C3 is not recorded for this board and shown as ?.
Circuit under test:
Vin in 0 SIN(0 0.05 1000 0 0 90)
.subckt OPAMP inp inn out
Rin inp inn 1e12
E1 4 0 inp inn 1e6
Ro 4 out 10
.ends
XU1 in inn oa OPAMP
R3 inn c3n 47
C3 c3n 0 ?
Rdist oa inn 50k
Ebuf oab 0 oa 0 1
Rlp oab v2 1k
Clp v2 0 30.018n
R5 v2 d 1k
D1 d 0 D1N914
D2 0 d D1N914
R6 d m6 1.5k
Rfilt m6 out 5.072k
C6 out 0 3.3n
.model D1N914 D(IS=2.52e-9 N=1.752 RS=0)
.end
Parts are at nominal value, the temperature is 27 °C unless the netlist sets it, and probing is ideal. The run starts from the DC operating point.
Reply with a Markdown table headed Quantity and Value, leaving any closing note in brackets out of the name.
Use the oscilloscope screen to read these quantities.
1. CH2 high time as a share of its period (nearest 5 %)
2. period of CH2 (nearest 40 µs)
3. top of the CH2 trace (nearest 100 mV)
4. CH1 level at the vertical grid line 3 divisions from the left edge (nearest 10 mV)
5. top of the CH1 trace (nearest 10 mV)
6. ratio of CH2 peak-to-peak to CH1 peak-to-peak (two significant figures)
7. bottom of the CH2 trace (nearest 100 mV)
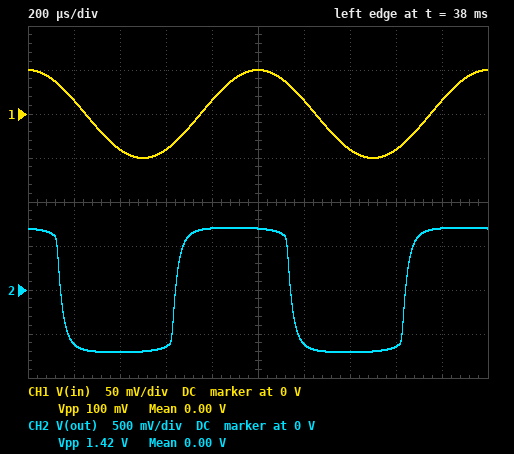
| Quantity | Value |
|---|---|
| CH2 high time as a share of its period | 50 % |
| period of CH2 | 1.00 ms |
| top of the CH2 trace | 700 mV |
| CH1 level at the vertical grid line 3 divisions from the left edge | -40 mV |
| top of the CH1 trace | 50 mV |
| ratio of CH2 peak-to-peak to CH1 peak-to-peak | 14 |
| bottom of the CH2 trace | -700 mV |
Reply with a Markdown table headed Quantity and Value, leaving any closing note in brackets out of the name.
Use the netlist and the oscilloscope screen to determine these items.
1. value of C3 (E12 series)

| Quantity | Value |
|---|---|
| value of C3 | 2.7 µF |
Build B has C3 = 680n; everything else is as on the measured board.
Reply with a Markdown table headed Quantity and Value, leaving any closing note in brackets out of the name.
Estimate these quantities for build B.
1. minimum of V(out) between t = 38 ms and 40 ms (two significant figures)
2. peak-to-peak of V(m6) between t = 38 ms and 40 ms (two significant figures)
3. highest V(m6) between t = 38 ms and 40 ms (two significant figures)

| Quantity | Value |
|---|---|
| minimum of V(out) between t = 38 ms and 40 ms | -660 mV |
| peak-to-peak of V(m6) between t = 38 ms and 40 ms | 1.3 V |
| highest V(m6) between t = 38 ms and 40 ms | 660 mV |
